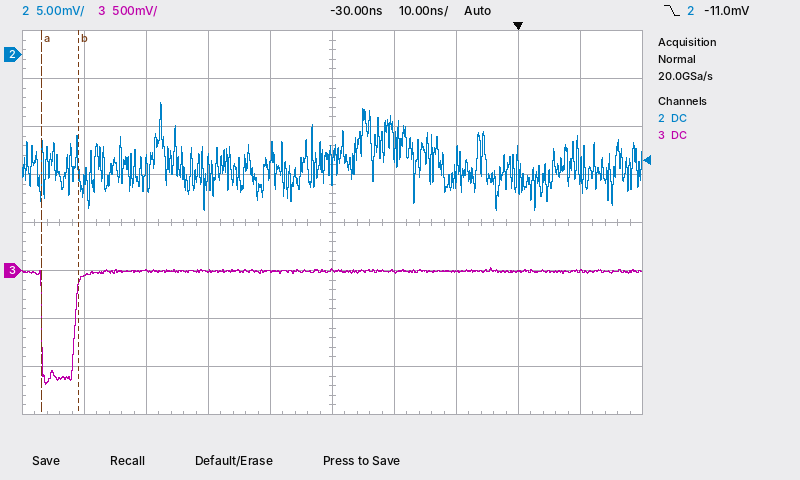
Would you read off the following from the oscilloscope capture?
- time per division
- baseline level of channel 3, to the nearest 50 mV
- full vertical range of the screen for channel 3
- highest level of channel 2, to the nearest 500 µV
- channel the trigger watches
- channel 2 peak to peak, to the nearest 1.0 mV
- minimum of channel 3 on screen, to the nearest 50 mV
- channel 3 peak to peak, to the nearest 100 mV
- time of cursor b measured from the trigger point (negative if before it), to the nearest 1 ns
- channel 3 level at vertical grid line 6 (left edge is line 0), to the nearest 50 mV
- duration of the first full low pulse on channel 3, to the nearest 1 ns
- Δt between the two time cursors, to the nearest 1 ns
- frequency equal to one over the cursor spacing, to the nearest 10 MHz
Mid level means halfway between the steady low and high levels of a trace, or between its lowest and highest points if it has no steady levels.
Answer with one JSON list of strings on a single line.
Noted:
["10 ns", "0 mV", "4 V", "-5.0 mV", "channel 2", "11.0 mV", "-1.20 V", "1.20 V", "-71 ns", "0 mV", "5 ns", "6 ns", "170 MHz"]
